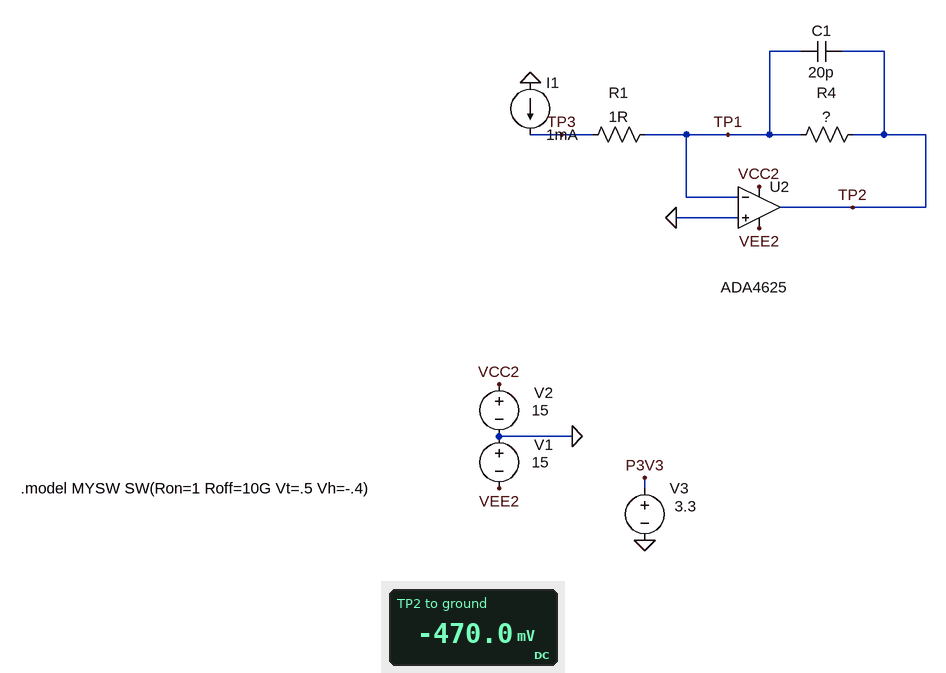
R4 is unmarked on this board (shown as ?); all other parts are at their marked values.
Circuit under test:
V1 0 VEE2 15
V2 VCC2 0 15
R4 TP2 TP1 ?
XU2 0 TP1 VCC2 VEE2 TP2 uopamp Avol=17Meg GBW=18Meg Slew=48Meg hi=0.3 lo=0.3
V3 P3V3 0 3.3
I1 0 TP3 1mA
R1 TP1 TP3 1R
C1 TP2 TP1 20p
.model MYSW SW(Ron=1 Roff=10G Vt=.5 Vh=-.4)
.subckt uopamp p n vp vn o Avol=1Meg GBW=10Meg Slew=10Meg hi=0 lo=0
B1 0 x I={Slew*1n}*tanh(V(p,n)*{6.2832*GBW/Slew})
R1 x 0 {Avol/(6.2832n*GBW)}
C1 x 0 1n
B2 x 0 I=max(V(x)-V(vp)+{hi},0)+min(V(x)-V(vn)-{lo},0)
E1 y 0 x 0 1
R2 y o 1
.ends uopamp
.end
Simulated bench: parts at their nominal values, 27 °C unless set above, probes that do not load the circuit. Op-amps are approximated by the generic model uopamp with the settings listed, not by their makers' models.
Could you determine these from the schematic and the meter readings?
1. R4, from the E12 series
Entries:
470 Ω
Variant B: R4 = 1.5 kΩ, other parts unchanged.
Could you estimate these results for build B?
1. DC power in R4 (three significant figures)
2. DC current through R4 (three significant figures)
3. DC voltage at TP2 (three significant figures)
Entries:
1.50 mW
1.00 mA
-1.50 V
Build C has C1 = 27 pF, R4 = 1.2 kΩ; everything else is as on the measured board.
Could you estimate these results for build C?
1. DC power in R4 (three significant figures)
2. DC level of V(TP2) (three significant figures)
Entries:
1.20 mW
-1.20 V
